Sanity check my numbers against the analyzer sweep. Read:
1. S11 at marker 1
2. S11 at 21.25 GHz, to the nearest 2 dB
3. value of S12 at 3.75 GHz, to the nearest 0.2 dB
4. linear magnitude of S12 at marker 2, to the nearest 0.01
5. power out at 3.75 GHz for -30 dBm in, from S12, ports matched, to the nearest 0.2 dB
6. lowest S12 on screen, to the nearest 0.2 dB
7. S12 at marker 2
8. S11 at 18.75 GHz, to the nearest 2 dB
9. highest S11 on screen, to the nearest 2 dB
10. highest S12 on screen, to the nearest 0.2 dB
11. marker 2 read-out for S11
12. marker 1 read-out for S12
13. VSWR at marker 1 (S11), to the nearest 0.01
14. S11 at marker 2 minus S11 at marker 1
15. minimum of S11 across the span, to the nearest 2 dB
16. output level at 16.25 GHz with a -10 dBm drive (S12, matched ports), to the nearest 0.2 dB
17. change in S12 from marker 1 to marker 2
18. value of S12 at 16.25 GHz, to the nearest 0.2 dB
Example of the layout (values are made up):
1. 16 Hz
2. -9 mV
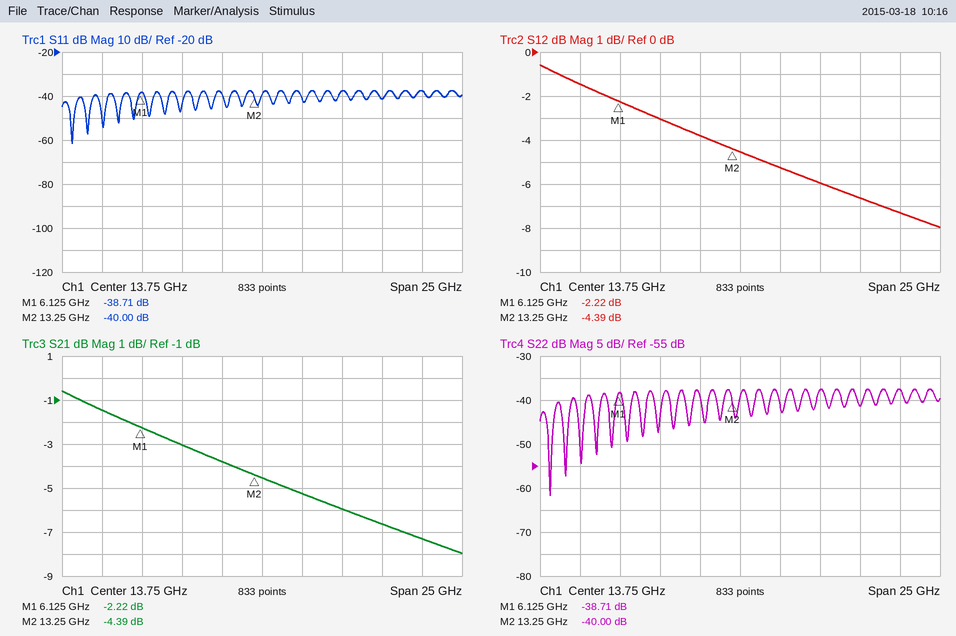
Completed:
1. -38.71 dB
2. -42 dB
3. -1.4 dB
4. 0.60
5. -31.4 dBm
6. -8.0 dB
7. -4.39 dB
8. -38 dB
9. -38 dB
10. -0.6 dB
11. -40.00 dB
12. -2.22 dB
13. 1.02
14. -1.29 dB
15. -62 dB
16. -15.2 dBm
17. -2.17 dB
18. -5.2 dB
